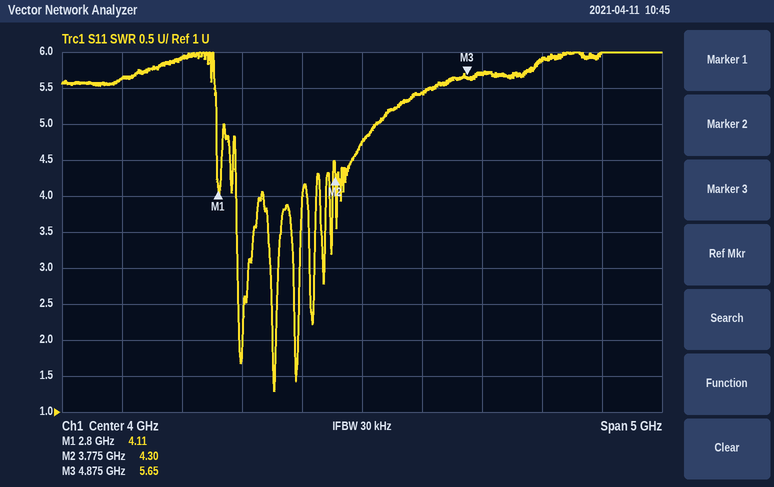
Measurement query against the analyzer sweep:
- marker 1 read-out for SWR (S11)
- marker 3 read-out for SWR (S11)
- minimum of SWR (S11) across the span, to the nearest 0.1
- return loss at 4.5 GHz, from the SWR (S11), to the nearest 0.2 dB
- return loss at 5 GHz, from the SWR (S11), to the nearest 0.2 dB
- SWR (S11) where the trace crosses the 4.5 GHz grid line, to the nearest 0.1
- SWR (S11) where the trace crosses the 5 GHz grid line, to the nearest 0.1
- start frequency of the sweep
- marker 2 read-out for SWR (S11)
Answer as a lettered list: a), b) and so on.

a) 4.11
b) 5.65
c) 1.3
d) 3.2 dB
e) 3.0 dB
f) 5.4
g) 5.7
h) 1.5 GHz
i) 4.30
